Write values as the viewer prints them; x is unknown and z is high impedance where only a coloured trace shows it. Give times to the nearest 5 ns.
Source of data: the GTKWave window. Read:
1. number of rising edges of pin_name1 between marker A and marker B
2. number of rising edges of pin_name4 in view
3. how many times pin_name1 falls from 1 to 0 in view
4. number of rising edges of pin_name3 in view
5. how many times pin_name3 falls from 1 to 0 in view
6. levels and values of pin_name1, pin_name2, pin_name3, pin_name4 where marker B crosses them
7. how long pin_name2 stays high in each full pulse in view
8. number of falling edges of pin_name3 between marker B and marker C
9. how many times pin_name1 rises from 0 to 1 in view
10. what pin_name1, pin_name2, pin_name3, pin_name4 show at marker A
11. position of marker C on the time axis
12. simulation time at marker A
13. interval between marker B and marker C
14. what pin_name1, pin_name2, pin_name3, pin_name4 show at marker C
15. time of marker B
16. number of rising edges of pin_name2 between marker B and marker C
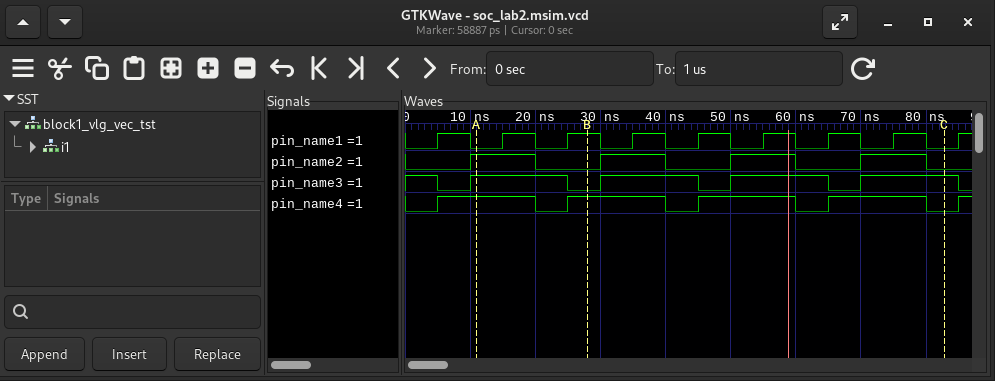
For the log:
2
5
8
4
5
pin_name1=1, pin_name2=0, pin_name3=0, pin_name4=1
10 ns, 10 ns, 10 ns, 10 ns
2
9
pin_name1=0, pin_name2=1, pin_name3=1, pin_name4=1
85 ns
10 ns
55 ns
pin_name1=0, pin_name2=0, pin_name3=1, pin_name4=0
30 ns
3
